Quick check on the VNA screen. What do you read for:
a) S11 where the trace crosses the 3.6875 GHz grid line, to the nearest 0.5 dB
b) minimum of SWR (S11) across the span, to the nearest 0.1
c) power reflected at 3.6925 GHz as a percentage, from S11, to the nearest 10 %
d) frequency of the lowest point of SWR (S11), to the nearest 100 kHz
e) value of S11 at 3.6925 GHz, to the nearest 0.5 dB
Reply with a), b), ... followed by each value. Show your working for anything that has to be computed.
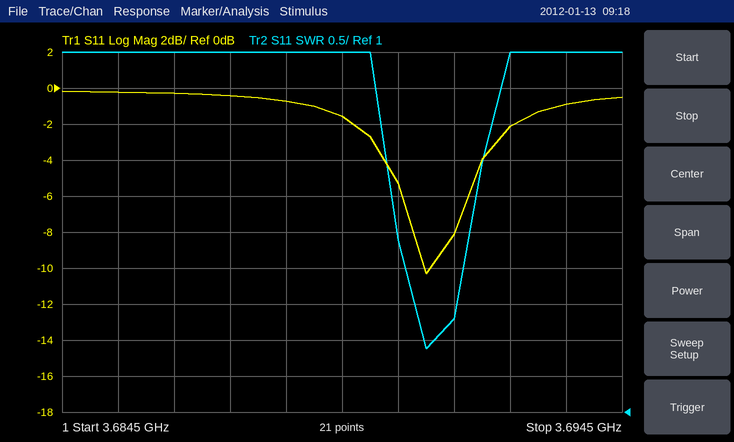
a) -0.5 dB
b) 1.9
c) 10^(-2/10) ≈ 63.1 %, so 60 % to the nearest 10 %
d) 3.6910 GHz
e) -2.0 dB
